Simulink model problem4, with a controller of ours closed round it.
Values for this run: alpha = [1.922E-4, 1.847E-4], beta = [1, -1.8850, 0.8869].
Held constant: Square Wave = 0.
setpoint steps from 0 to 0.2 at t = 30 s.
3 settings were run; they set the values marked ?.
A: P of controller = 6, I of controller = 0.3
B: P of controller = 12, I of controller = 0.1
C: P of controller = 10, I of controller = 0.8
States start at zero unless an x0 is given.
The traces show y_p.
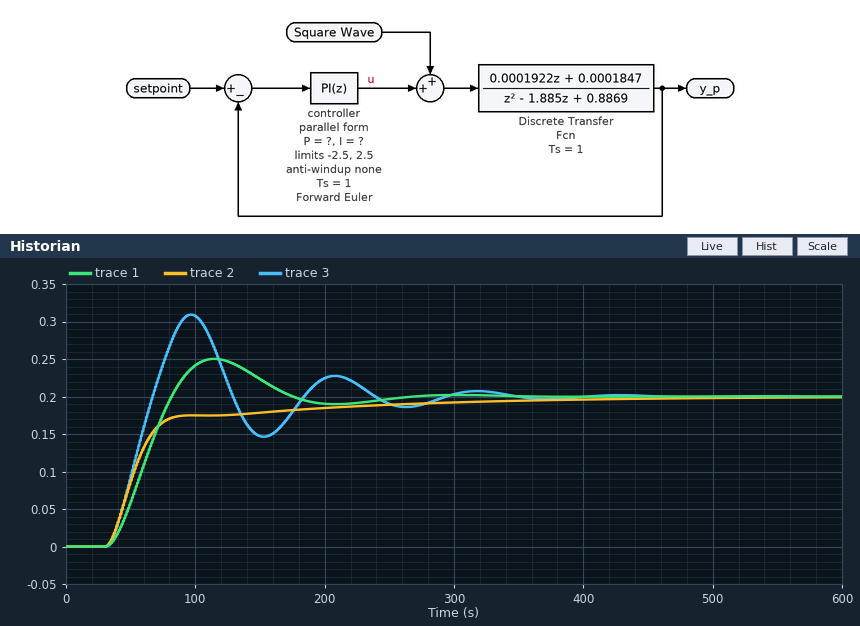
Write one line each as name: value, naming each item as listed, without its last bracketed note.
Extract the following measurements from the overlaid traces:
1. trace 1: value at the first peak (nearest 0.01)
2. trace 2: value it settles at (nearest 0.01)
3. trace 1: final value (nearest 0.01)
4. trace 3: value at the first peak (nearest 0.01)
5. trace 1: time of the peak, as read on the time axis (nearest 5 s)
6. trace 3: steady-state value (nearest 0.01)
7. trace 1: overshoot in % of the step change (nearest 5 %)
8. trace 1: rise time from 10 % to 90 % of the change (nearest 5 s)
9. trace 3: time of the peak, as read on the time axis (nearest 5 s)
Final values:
trace 1: value at the first peak: 0.25
trace 2: value it settles at: 0.20
trace 1: final value: 0.20
trace 3: value at the first peak: 0.31
trace 1: time of the peak, as read on the time axis: 115 s
trace 3: steady-state value: 0.20
trace 1: overshoot in % of the step change: 25 %
trace 1: rise time from 10 % to 90 % of the change: 35 s
trace 3: time of the peak, as read on the time axis: 95 s
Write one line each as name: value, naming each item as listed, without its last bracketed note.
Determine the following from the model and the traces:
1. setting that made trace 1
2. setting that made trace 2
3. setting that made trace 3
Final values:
setting that made trace 1: A
setting that made trace 2: B
setting that made trace 3: C
